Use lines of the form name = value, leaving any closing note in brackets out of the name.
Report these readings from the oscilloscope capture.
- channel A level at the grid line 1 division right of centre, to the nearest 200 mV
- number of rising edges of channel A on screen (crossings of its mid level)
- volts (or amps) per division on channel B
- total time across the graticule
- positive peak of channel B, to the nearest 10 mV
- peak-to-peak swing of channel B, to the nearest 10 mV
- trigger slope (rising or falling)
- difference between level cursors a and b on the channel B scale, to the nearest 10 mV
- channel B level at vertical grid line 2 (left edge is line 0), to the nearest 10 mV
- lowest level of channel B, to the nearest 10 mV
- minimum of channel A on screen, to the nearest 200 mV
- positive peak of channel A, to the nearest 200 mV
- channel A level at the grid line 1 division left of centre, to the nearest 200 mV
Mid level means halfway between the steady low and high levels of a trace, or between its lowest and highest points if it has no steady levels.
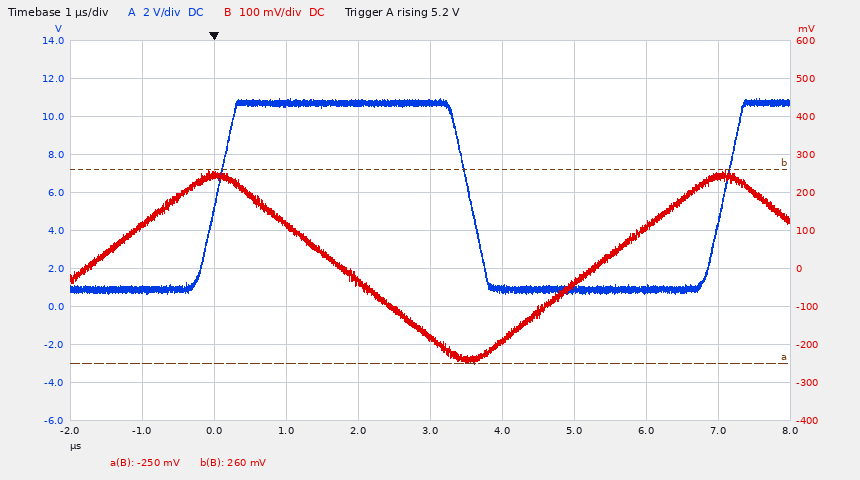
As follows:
channel A level at the grid line 1 division right of centre, to the nearest 200 mV = 1.0 V
number of rising edges of channel A on screen = 2
volts (or amps) per division on channel B = 100 mV
total time across the graticule = 10 µs
positive peak of channel B, to the nearest 10 mV = 260 mV
peak-to-peak swing of channel B, to the nearest 10 mV = 510 mV
trigger slope = rising
difference between level cursors a and b on the channel B scale, to the nearest 10 mV = 510 mV
channel B level at vertical grid line 2 (left edge is line 0), to the nearest 10 mV = 250 mV
lowest level of channel B, to the nearest 10 mV = -250 mV
minimum of channel A on screen, to the nearest 200 mV = 600 mV
positive peak of channel A, to the nearest 200 mV = 11.0 V
channel A level at the grid line 1 division left of centre, to the nearest 200 mV = 10.8 V
